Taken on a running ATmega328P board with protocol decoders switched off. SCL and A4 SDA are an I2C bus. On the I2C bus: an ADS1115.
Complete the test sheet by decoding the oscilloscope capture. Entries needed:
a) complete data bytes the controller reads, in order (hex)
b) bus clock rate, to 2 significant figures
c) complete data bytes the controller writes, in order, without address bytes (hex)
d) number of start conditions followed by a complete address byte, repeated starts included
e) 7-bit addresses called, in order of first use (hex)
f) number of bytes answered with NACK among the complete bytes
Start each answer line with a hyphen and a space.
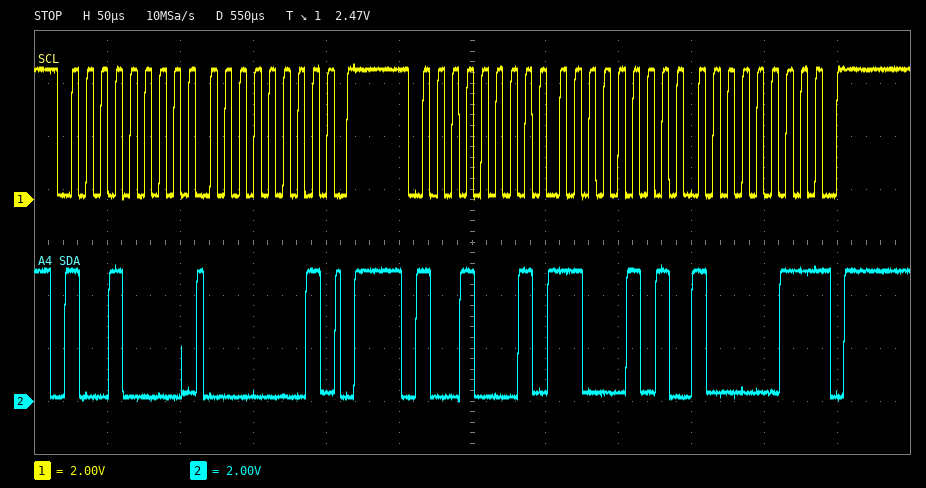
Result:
- C5 83
- 100 kHz
- 01
- 2
- 0x48
- 1
